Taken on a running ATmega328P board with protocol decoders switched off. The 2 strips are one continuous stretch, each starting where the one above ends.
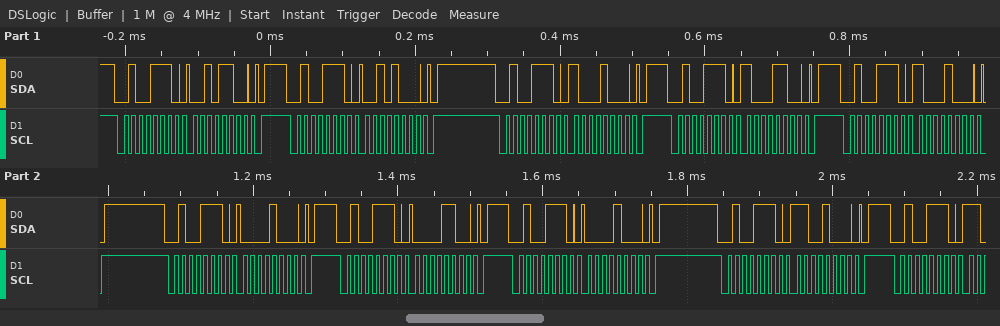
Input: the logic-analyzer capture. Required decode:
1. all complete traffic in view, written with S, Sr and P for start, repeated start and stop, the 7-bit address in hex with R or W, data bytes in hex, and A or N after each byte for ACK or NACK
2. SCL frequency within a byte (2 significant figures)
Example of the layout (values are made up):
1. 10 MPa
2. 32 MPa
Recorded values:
1. S 27W A 2C A P S 27W A 28 A P S 27W A 88 A P S 27W A 8C A P S 27W A 88 A P S 27W A 08 A P S 27W A 0C A P S 27W A 08 A P S 27W A C8 A P S 27W A
2. 100 kHz
